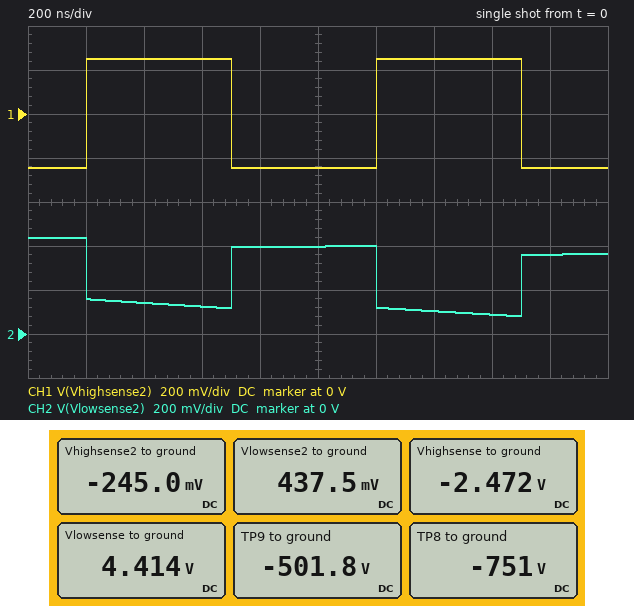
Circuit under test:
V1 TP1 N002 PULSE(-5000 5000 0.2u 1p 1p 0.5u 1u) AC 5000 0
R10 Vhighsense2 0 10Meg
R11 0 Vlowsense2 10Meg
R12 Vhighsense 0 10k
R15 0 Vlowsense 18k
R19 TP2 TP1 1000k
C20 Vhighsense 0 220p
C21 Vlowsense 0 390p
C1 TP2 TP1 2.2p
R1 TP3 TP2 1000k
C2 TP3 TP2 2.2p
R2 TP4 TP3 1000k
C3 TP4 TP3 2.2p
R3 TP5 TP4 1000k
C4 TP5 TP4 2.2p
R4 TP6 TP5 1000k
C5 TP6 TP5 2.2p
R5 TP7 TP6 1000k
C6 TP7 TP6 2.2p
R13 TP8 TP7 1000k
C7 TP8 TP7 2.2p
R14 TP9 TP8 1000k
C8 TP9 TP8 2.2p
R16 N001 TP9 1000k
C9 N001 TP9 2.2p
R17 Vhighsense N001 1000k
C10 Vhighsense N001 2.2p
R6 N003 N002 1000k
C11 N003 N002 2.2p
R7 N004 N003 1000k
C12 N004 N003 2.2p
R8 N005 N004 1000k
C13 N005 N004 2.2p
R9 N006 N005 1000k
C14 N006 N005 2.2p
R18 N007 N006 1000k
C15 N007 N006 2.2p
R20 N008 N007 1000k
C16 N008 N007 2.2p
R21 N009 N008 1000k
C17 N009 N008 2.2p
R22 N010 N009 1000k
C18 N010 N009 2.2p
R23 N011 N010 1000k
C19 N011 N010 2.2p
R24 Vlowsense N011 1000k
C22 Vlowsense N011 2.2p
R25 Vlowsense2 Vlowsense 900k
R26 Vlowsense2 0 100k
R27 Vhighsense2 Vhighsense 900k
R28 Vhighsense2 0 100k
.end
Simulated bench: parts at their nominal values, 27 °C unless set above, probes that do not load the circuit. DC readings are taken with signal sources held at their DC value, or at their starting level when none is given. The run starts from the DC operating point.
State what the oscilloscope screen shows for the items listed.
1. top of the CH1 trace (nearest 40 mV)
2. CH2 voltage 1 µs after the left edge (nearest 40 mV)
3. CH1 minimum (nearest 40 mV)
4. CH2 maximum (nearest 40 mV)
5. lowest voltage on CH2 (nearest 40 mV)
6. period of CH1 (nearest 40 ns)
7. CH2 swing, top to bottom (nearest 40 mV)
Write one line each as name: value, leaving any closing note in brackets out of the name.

top of the CH1 trace: 240 mV
CH2 voltage 1 µs after the left edge: 400 mV
CH1 minimum: -240 mV
CH2 maximum: 440 mV
lowest voltage on CH2: 80 mV
period of CH1: 1.00 µs
CH2 swing, top to bottom: 360 mV
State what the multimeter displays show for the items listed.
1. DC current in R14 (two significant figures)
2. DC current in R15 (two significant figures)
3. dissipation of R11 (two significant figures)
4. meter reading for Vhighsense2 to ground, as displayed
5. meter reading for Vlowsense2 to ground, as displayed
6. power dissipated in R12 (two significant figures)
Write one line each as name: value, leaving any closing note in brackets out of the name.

DC current in R14: 250 µA
DC current in R15: 250 µA
dissipation of R11: 19 nW
meter reading for Vhighsense2 to ground, as displayed: -245.0 mV
meter reading for Vlowsense2 to ground, as displayed: 437.5 mV
power dissipated in R12: 610 µW
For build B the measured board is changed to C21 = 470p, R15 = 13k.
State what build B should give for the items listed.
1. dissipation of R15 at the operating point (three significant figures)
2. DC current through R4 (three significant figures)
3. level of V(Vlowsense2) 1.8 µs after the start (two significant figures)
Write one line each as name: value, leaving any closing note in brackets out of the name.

dissipation of R15 at the operating point: 790 µW
DC current through R4: 250 µA
level of V(Vlowsense2) 1.8 µs after the start: 260 mV
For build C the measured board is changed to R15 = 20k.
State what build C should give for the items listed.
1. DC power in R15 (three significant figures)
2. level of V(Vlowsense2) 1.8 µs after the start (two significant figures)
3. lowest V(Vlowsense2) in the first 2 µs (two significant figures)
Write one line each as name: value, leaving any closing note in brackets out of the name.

DC power in R15: 1.20 mW
level of V(Vlowsense2) 1.8 µs after the start: 400 mV
lowest V(Vlowsense2) in the first 2 µs: 120 mV
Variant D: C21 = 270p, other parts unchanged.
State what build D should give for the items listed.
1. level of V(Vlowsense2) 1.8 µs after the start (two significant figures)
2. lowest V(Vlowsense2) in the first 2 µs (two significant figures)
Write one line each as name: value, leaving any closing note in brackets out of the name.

level of V(Vlowsense2) 1.8 µs after the start: 350 mV
lowest V(Vlowsense2) in the first 2 µs: -51 mV
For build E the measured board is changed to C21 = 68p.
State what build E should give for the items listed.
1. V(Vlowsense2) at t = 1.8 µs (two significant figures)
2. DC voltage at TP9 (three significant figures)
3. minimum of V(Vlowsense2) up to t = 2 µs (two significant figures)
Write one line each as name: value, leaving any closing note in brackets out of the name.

V(Vlowsense2) at t = 1.8 µs: 760 mV
DC voltage at TP9: -502 V
minimum of V(Vlowsense2) up to t = 2 µs: -1.2 V
